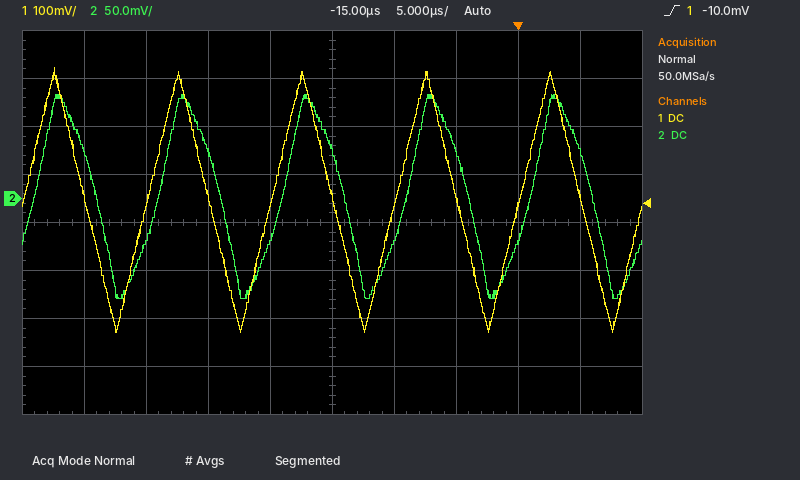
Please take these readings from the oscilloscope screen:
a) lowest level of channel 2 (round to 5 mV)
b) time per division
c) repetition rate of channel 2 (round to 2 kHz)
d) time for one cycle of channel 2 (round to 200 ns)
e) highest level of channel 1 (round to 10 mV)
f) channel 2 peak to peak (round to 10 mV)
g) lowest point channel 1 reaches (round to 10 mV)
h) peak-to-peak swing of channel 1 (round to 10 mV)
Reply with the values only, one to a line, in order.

-105 mV
5 µs
100 kHz
10.0 µs
270 mV
210 mV
-280 mV
550 mV
